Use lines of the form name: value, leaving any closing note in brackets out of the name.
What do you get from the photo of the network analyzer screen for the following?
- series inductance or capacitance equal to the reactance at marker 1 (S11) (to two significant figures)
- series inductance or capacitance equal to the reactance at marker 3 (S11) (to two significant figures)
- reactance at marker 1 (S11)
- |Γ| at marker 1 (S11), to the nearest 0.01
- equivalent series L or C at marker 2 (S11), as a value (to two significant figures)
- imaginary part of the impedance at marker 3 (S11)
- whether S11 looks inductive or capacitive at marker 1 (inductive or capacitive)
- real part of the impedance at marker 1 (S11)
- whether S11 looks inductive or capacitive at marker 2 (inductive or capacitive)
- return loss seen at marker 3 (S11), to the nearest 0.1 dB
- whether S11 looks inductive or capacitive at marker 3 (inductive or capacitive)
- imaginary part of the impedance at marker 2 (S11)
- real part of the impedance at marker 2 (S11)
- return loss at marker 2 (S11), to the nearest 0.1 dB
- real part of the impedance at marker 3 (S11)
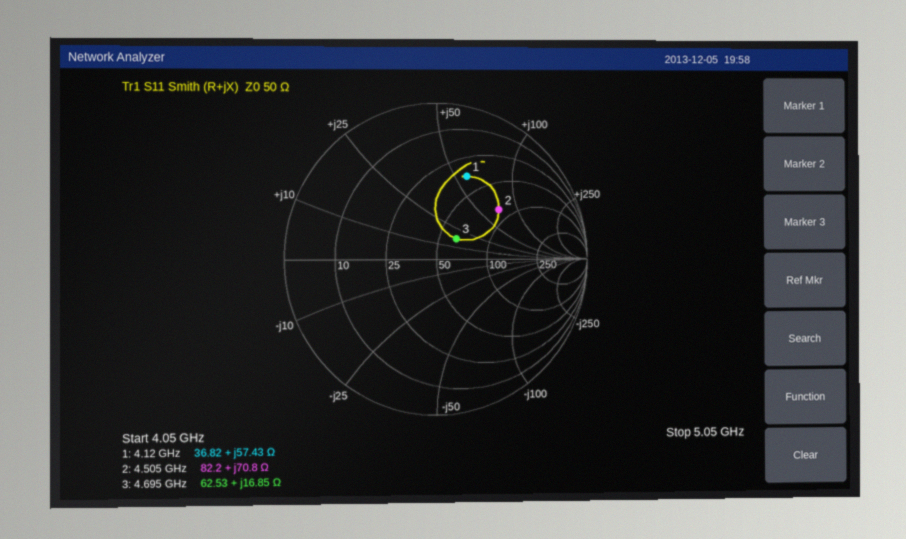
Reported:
series inductance or capacitance equal to the reactance at marker 1 (S11): 2.2 nH
series inductance or capacitance equal to the reactance at marker 3 (S11): 570 pH
reactance at marker 1: +57.43 Ω
|Γ| at marker 1 (S11), to the nearest 0.01: 0.57
equivalent series L or C at marker 2 (S11), as a value: 2.5 nH
imaginary part of the impedance at marker 3: +16.85 Ω
whether S11 looks inductive or capacitive at marker 1: inductive
real part of the impedance at marker 1: 36.82 Ω
whether S11 looks inductive or capacitive at marker 2: inductive
return loss seen at marker 3 (S11), to the nearest 0.1 dB: 14.7 dB
whether S11 looks inductive or capacitive at marker 3: inductive
imaginary part of the impedance at marker 2: +70.8 Ω
real part of the impedance at marker 2: 82.2 Ω
return loss at marker 2 (S11), to the nearest 0.1 dB: 5.7 dB
real part of the impedance at marker 3: 62.53 Ω
